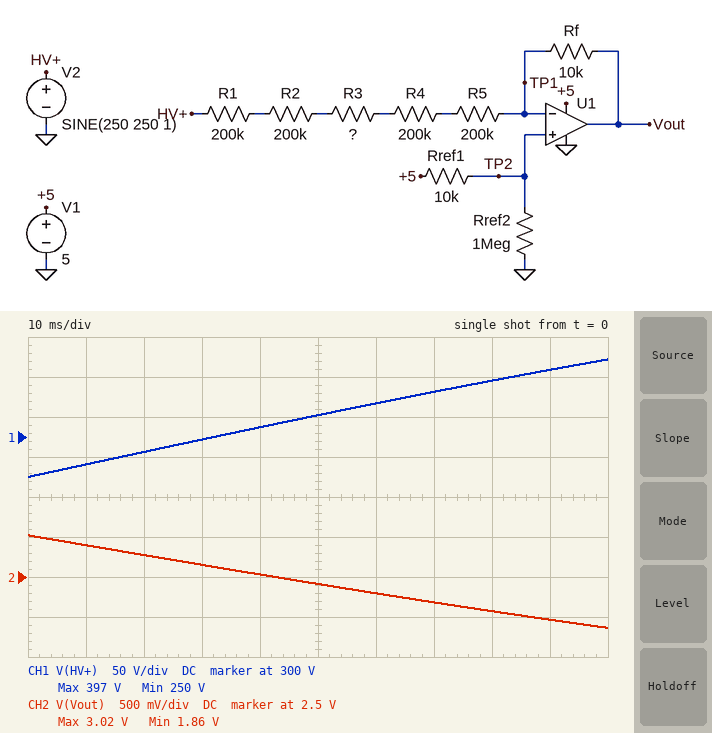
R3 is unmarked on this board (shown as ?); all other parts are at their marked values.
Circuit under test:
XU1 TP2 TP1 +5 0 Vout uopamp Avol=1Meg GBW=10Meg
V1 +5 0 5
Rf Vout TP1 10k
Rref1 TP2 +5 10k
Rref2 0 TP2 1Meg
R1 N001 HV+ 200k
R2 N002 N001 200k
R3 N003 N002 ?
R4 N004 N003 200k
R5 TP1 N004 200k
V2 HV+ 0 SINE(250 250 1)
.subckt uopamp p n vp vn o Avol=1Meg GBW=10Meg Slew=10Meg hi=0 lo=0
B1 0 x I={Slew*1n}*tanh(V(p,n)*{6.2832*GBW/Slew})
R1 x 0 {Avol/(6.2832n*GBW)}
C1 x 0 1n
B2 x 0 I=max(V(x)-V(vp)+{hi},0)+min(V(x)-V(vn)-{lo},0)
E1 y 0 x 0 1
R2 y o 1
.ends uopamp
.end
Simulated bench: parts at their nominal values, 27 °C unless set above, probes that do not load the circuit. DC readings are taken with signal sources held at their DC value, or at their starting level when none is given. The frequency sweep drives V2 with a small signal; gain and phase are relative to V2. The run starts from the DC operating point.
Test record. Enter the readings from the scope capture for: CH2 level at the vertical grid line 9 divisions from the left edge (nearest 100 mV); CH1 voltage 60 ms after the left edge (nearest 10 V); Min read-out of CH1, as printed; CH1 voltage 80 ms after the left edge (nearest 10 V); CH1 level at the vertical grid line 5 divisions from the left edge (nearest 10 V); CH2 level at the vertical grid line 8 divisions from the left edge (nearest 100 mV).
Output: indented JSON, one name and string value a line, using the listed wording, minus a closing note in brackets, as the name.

{
  "CH2 level at the vertical grid line 9 divisions from the left edge": "2.0 V",
  "CH1 voltage 60 ms after the left edge": "340 V",
  "Min read-out of CH1, as printed": "250 V",
  "CH1 voltage 80 ms after the left edge": "370 V",
  "CH1 level at the vertical grid line 5 divisions from the left edge": "330 V",
  "CH2 level at the vertical grid line 8 divisions from the left edge": "2.1 V"
}
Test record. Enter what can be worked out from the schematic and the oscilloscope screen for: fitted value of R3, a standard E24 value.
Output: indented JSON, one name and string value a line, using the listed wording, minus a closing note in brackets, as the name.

{
  "fitted value of R3, a standard E24 value": "470 kΩ"
}
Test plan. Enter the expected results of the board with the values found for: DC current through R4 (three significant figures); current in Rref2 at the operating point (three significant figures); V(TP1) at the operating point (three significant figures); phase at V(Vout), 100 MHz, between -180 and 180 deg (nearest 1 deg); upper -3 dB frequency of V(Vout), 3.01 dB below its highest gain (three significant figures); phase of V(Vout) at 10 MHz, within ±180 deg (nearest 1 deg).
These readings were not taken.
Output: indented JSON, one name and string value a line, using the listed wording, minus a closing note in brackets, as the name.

{
  "DC current through R4": "193 µA",
  "current in Rref2 at the operating point": "4.95 µA",
  "V(TP1) at the operating point": "4.95 V",
  "phase at V(Vout), 100 MHz, between -180 and 180 deg": "96 deg",
  "upper -3 dB frequency of V(Vout), 3.01 dB below its highest gain": "9.92 MHz",
  "phase of V(Vout) at 10 MHz, within ±180 deg": "135 deg"
}
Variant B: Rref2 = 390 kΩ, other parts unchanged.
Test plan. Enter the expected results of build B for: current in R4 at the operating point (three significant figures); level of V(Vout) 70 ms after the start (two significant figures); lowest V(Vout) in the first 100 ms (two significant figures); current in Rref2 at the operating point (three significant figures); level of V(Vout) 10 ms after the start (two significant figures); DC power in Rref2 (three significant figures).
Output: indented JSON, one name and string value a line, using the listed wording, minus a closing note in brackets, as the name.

{
  "current in R4 at the operating point": "193 µA",
  "level of V(Vout) 70 ms after the start": "2.1 V",
  "lowest V(Vout) in the first 100 ms": "1.8 V",
  "current in Rref2 at the operating point": "12.5 µA",
  "level of V(Vout) 10 ms after the start": "2.8 V",
  "DC power in Rref2": "60.9 µW"
}
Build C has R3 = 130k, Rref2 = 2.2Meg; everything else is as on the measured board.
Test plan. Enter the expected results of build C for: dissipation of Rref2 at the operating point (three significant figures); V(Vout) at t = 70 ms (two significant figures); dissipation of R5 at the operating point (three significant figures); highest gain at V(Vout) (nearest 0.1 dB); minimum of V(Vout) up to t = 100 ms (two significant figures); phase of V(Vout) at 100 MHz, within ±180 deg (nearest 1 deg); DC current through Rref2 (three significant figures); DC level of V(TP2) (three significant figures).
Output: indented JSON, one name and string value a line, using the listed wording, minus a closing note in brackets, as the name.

{
  "dissipation of Rref2 at the operating point": "11.3 µW",
  "V(Vout) at t = 70 ms": "1.2 V",
  "dissipation of R5 at the operating point": "13.9 mW",
  "highest gain at V(Vout)": "-39.4 dB",
  "minimum of V(Vout) up to t = 100 ms": "760 mV",
  "phase of V(Vout) at 100 MHz, within ±180 deg": "96 deg",
  "DC current through Rref2": "2.26 µA",
  "DC level of V(TP2)": "4.98 V"
}
